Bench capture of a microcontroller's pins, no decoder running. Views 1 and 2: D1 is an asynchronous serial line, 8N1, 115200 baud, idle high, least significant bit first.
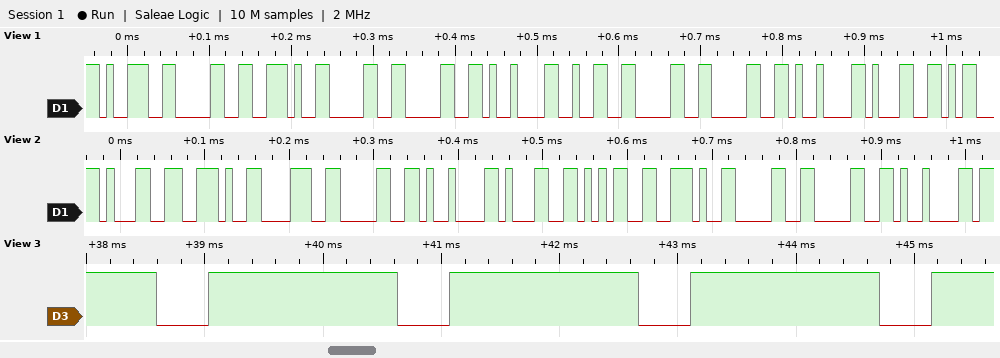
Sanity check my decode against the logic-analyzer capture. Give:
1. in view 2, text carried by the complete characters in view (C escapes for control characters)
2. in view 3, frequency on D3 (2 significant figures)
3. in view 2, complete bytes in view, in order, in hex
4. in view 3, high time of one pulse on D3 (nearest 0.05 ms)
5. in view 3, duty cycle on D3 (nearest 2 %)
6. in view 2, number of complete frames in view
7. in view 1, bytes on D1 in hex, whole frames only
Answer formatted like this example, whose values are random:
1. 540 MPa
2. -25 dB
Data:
1. "1.80\t15.00\t"
2. 490 Hz
3. 0x31 0x2E 0x38 0x30 0x09 0x31 0x35 0x2E 0x30 0x30 0x09
4. 1.60 ms
5. 78 %
6. 11
7. 39 30 2E 30 30 09 32 30 30 09 31
